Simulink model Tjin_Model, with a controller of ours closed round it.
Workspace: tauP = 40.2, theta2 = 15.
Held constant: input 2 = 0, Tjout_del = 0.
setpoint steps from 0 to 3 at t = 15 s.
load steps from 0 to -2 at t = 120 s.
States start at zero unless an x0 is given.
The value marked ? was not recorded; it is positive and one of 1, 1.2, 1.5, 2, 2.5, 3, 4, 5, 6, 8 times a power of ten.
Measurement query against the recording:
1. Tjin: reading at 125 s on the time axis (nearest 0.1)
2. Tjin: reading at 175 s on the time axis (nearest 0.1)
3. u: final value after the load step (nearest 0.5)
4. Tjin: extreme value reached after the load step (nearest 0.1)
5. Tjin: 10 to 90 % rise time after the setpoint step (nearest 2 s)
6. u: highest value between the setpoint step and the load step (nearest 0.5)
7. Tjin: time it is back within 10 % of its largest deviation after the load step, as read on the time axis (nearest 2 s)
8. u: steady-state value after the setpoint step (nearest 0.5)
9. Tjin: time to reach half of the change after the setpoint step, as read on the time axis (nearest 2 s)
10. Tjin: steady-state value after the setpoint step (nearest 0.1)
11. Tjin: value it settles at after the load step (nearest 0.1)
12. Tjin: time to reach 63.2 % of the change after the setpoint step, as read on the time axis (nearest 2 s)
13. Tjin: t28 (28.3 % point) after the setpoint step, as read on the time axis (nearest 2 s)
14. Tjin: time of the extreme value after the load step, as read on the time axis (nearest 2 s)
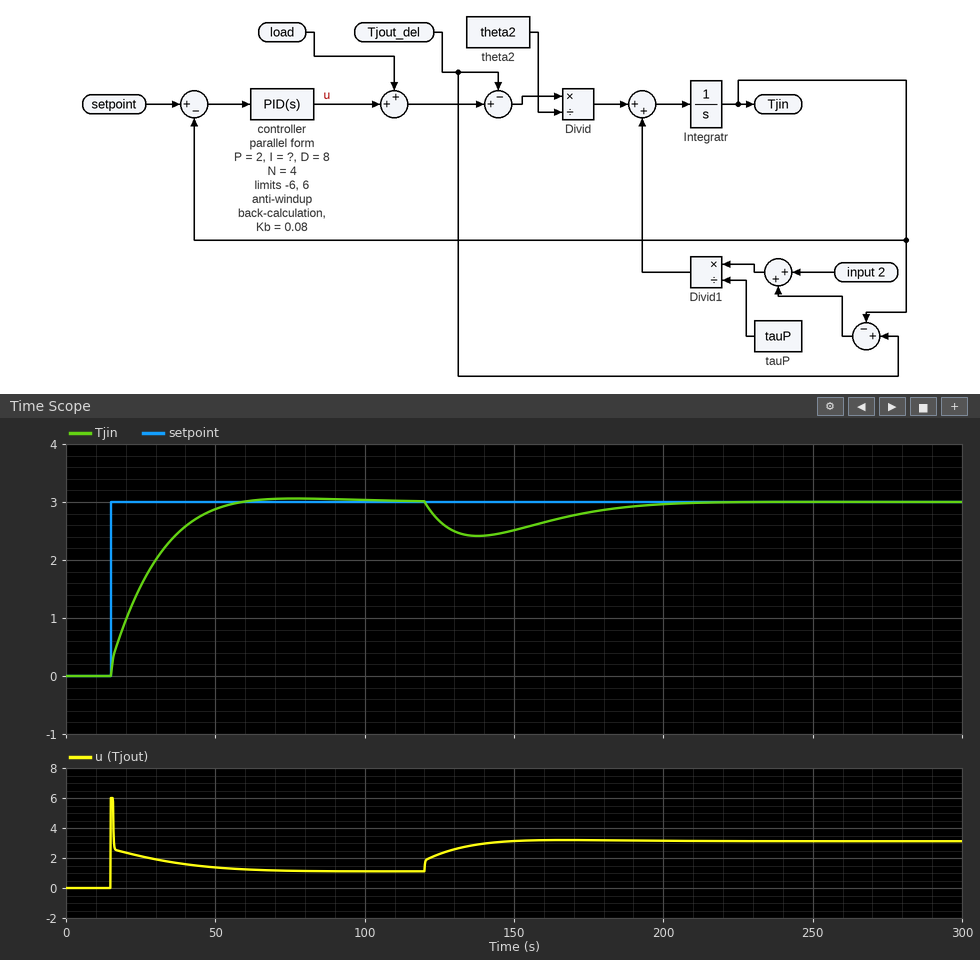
2.7
2.8
3.0
2.4
28 s
6.0
194 s
1.0
24 s
3.0
3.0
28 s
20 s
138 s
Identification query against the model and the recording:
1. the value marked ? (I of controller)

0.08
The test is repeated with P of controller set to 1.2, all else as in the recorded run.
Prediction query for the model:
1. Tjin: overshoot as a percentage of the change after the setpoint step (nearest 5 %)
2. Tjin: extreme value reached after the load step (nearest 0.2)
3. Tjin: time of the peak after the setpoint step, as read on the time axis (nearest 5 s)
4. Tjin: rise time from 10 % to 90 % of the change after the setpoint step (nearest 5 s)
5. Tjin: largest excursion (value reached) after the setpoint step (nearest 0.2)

10 %
2.2
70 s
30 s
3.4
